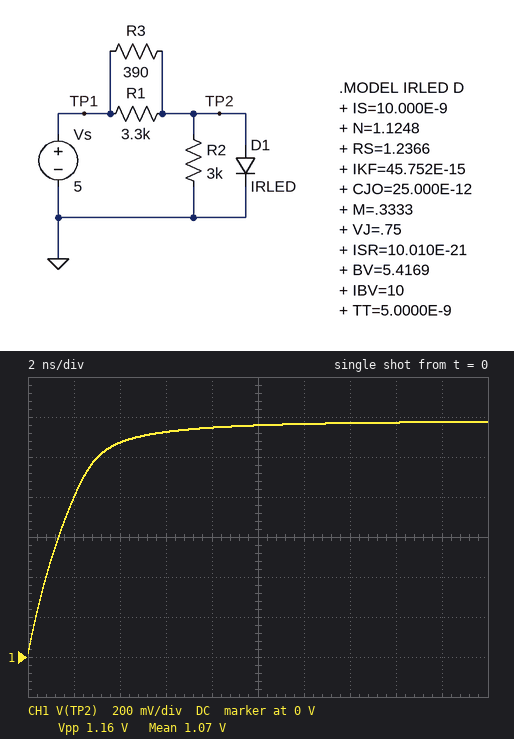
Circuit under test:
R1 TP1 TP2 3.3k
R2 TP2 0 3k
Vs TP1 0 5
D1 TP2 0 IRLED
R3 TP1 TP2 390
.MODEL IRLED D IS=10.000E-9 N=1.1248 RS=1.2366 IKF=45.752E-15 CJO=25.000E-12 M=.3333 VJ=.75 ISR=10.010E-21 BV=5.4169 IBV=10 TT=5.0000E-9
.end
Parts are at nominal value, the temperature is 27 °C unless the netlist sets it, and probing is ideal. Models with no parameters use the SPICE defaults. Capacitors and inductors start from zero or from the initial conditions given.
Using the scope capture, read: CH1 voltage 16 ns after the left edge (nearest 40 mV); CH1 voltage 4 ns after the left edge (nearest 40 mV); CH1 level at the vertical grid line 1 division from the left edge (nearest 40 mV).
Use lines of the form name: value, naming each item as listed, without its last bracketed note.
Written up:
CH1 voltage 16 ns after the left edge: 1.16 V
CH1 voltage 4 ns after the left edge: 1.08 V
CH1 level at the vertical grid line 1 division from the left edge: 800 mV
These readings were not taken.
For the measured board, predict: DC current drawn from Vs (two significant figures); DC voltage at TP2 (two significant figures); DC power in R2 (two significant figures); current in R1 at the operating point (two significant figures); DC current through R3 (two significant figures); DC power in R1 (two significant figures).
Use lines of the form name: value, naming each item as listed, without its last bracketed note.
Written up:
DC current drawn from Vs: 11 mA
DC voltage at TP2: 1.2 V
DC power in R2: 460 µW
current in R1 at the operating point: 1.2 mA
DC current through R3: 9.8 mA
DC power in R1: 4.4 mW
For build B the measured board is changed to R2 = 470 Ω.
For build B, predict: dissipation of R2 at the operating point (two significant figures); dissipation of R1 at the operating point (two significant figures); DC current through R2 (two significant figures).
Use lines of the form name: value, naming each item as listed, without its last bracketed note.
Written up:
dissipation of R2 at the operating point: 2.9 mW
dissipation of R1 at the operating point: 4.5 mW
DC current through R2: 2.5 mA
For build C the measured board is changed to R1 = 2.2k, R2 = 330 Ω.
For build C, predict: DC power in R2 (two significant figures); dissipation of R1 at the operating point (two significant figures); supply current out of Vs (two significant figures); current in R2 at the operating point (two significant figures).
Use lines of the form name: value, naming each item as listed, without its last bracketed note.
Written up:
DC power in R2: 4.1 mW
dissipation of R1 at the operating point: 6.7 mW
supply current out of Vs: 12 mA
current in R2 at the operating point: 3.5 mA
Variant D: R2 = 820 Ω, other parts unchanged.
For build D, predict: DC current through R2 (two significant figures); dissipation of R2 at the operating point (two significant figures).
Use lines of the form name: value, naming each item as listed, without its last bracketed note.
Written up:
DC current through R2: 1.4 mA
dissipation of R2 at the operating point: 1.7 mW
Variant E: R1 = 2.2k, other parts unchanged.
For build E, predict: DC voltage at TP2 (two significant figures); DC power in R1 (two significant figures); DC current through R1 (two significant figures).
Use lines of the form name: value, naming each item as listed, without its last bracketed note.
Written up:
DC voltage at TP2: 1.2 V
DC power in R1: 6.6 mW
DC current through R1: 1.7 mA
